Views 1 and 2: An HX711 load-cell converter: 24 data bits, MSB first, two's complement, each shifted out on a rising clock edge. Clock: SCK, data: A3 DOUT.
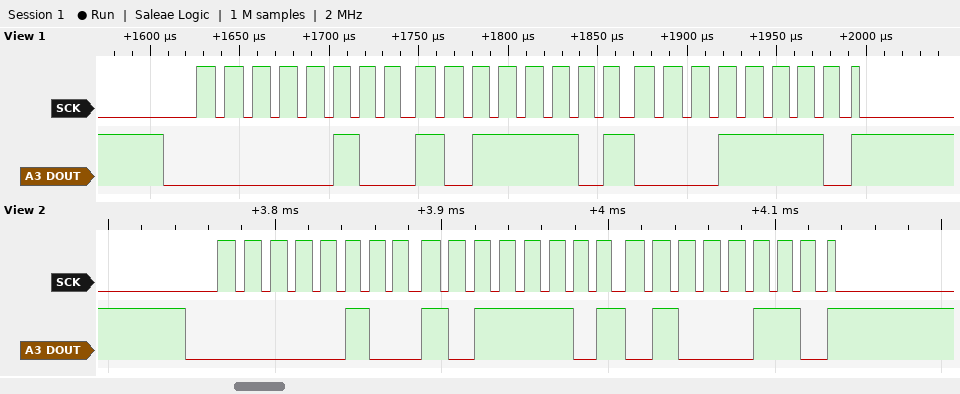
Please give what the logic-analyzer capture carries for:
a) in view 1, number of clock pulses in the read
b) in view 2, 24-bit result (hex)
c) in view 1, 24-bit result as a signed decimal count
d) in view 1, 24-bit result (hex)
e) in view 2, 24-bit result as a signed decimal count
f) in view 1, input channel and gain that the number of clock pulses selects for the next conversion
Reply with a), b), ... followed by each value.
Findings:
a) 25
b) 0x04BD46
c) 310558
d) 0x04BD1E
e) 310598
f) channel A, gain 128
